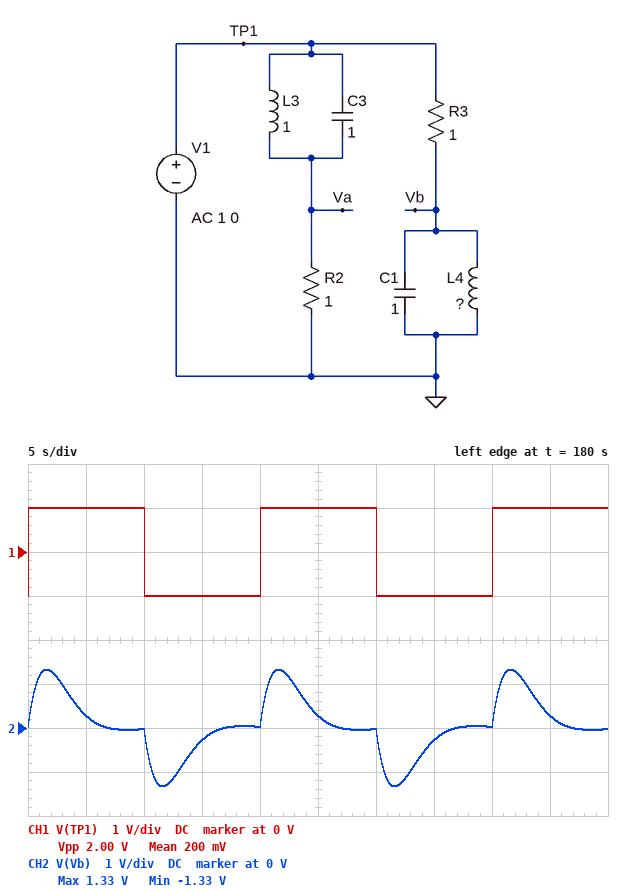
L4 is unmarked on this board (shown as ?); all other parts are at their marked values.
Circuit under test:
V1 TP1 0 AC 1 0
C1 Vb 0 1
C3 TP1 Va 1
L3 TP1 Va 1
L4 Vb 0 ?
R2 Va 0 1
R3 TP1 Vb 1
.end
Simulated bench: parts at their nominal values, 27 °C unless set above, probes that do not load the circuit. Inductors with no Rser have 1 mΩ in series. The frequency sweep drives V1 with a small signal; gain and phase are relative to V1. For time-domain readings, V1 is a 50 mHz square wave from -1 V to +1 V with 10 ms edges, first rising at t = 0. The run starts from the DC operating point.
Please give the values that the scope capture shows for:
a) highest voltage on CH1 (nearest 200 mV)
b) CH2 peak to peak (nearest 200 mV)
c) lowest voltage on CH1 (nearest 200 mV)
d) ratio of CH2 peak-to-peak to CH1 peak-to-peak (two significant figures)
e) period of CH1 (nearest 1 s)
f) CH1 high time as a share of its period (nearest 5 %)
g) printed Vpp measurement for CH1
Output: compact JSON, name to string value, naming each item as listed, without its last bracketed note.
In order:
{"highest voltage on CH1": "1.0 V", "CH2 peak to peak": "2.6 V", "lowest voltage on CH1": "-1.0 V", "ratio of CH2 peak-to-peak to CH1 peak-to-peak": "1.3", "period of CH1": "20 s", "CH1 high time as a share of its period": "50 %", "printed Vpp measurement for CH1": "2.00 V"}
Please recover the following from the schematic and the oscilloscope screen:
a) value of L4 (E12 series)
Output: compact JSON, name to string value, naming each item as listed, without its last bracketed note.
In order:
{"value of L4": "2.2 H"}
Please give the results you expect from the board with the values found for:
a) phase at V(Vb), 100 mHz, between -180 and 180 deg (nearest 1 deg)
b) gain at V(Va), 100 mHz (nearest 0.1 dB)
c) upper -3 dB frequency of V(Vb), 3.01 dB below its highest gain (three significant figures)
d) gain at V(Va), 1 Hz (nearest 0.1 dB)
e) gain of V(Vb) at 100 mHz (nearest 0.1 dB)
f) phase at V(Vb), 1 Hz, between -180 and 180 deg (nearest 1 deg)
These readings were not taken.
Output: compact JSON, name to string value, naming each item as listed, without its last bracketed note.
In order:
{"phase at V(Vb), 100 mHz, between -180 and 180 deg": "5 deg", "gain at V(Va), 100 mHz": "-3.2 dB", "upper -3 dB frequency of V(Vb), 3.01 dB below its highest gain": "213 mHz", "gain at V(Va), 1 Hz": "-0.1 dB", "gain of V(Vb) at 100 mHz": "0 dB", "phase at V(Vb), 1 Hz, between -180 and 180 deg": "-81 deg"}
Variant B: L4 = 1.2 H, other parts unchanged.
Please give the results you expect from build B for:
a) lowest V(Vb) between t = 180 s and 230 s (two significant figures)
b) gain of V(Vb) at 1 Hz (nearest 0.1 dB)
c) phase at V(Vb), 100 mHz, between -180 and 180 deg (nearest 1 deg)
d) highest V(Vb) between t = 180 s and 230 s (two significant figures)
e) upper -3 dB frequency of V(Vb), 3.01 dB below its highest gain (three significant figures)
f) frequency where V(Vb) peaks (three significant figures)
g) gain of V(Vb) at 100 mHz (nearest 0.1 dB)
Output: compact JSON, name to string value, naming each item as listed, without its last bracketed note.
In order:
{"lowest V(Vb) between t = 180 s and 230 s": "-1.1 V", "gain of V(Vb) at 1 Hz": "-15.9 dB", "phase at V(Vb), 100 mHz, between -180 and 180 deg": "35 deg", "highest V(Vb) between t = 180 s and 230 s": "1.1 V", "upper -3 dB frequency of V(Vb), 3.01 dB below its highest gain": "245 mHz", "frequency where V(Vb) peaks": "145 mHz", "gain of V(Vb) at 100 mHz": "-1.7 dB"}
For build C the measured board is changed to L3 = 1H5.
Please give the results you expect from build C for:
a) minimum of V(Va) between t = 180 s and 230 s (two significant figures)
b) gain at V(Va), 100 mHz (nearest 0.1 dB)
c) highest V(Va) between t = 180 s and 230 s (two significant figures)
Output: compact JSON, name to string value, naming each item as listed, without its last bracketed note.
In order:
{"minimum of V(Va) between t = 180 s and 230 s": "-1.1 V", "gain at V(Va), 100 mHz": "-8.0 dB", "highest V(Va) between t = 180 s and 230 s": "1.1 V"}
